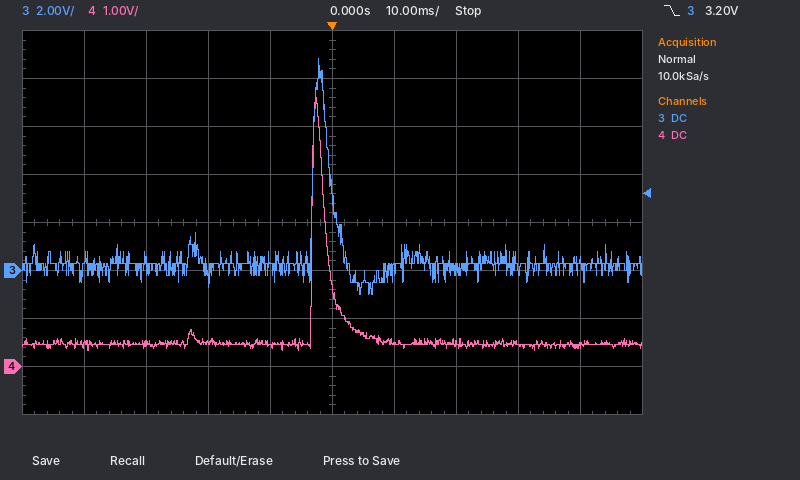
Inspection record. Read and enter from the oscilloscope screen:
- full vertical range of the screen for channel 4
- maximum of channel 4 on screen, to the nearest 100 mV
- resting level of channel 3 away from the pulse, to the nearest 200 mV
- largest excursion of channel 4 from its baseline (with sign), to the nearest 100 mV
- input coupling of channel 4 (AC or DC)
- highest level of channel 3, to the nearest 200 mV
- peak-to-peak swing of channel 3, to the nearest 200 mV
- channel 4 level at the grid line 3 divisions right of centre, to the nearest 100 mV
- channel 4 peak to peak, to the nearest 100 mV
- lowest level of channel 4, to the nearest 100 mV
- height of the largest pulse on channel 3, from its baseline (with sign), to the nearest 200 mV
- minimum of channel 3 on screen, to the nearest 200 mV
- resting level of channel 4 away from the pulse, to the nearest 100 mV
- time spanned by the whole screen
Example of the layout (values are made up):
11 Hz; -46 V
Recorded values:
8 V; 5.6 V; 200 mV; +5.1 V; DC; 8.8 V; 9.8 V; 500 mV; 5.3 V; 300 mV; +8.6 V; -1.0 V; 500 mV; 100 ms
